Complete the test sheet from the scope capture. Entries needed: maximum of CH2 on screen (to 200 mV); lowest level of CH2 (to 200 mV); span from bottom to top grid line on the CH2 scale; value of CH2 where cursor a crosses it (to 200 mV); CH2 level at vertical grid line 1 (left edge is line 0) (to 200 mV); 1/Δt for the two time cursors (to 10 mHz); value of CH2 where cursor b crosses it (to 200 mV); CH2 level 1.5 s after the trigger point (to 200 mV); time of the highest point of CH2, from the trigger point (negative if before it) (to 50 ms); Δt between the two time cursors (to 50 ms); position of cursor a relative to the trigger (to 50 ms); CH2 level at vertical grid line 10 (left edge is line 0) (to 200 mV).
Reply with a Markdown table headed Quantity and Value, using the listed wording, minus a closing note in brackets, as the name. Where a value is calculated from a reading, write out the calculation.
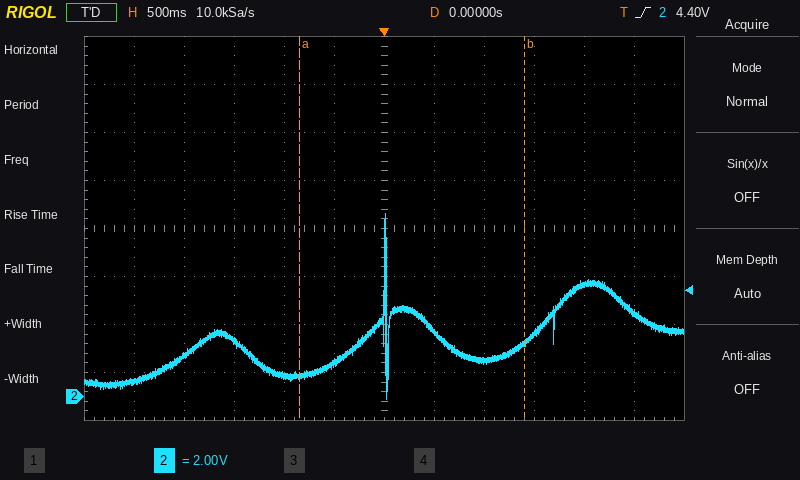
| Quantity | Value |
|---|---|
| maximum of CH2 on screen | 7.6 V |
| lowest level of CH2 | 0.0 V |
| span from bottom to top grid line on the CH2 scale | 16 V |
| value of CH2 where cursor a crosses it | 800 mV |
| CH2 level at vertical grid line 1 (left edge is line 0) | 600 mV |
| 1/Δt for the two time cursors | 1 / 2.25 s ≈ 440 mHz |
| value of CH2 where cursor b crosses it | 2.2 V |
| CH2 level 1.5 s after the trigger point | 2.6 V |
| time of the highest point of CH2, from the trigger point (negative if before it) | 0 ms |
| Δt between the two time cursors | 2.25 s |
| position of cursor a relative to the trigger | -850 ms |
| CH2 level at vertical grid line 10 (left edge is line 0) | 4.6 V |
